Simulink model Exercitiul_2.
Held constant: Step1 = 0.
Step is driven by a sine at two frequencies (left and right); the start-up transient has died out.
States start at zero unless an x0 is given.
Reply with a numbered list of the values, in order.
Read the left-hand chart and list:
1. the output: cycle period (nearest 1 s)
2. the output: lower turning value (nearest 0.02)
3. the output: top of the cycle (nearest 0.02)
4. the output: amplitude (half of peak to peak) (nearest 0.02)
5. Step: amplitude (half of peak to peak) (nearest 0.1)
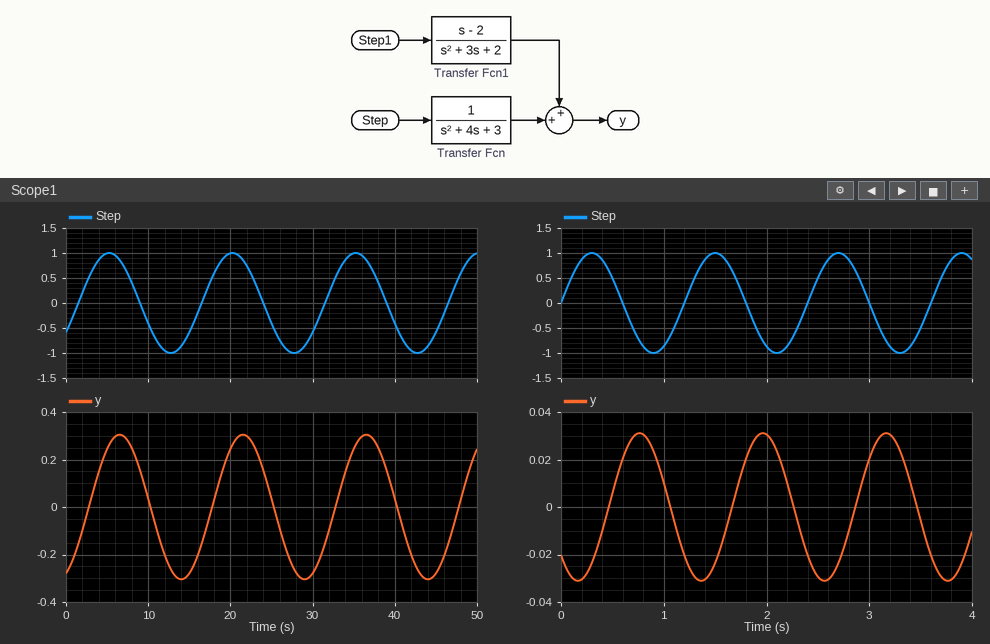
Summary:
1. 15 s
2. -0.30
3. 0.30
4. 0.30
5. 1.0
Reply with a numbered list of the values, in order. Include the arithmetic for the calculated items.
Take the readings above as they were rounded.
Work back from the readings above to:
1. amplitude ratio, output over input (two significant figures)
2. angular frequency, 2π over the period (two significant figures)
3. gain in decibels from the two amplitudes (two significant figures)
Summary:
1. 0.3 / 1 = 0.30
2. 2π / 15 = 0.42 rad/s
3. 20 log10(0.3 / 1) = -10 dB
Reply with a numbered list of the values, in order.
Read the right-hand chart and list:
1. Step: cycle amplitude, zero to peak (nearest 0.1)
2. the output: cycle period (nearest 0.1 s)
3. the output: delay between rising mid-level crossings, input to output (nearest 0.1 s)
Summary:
1. 1.0
2. 1.2 s
3. 0.5 s
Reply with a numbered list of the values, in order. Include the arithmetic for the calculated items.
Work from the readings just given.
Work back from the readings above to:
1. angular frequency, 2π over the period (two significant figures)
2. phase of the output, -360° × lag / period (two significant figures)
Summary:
1. 2π / 1.2 = 5.2 rad/s
2. -360 × 0.5 / 1.2 = -150°
